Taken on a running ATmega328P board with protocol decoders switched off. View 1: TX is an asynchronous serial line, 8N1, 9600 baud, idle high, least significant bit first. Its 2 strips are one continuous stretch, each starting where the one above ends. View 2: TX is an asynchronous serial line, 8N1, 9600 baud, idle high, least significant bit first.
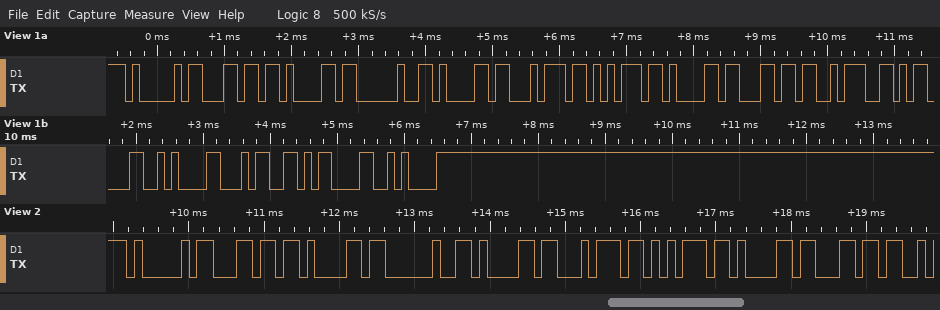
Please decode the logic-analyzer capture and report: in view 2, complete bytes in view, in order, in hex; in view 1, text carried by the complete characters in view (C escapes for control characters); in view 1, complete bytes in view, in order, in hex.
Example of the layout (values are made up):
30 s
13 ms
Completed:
41 6C 61 20 61 74 75 61 6C
"Ala atual:\r\n4\r\n"
41 6C 61 20 61 74 75 61 6C 3A 0D 0A 34 0D 0A
